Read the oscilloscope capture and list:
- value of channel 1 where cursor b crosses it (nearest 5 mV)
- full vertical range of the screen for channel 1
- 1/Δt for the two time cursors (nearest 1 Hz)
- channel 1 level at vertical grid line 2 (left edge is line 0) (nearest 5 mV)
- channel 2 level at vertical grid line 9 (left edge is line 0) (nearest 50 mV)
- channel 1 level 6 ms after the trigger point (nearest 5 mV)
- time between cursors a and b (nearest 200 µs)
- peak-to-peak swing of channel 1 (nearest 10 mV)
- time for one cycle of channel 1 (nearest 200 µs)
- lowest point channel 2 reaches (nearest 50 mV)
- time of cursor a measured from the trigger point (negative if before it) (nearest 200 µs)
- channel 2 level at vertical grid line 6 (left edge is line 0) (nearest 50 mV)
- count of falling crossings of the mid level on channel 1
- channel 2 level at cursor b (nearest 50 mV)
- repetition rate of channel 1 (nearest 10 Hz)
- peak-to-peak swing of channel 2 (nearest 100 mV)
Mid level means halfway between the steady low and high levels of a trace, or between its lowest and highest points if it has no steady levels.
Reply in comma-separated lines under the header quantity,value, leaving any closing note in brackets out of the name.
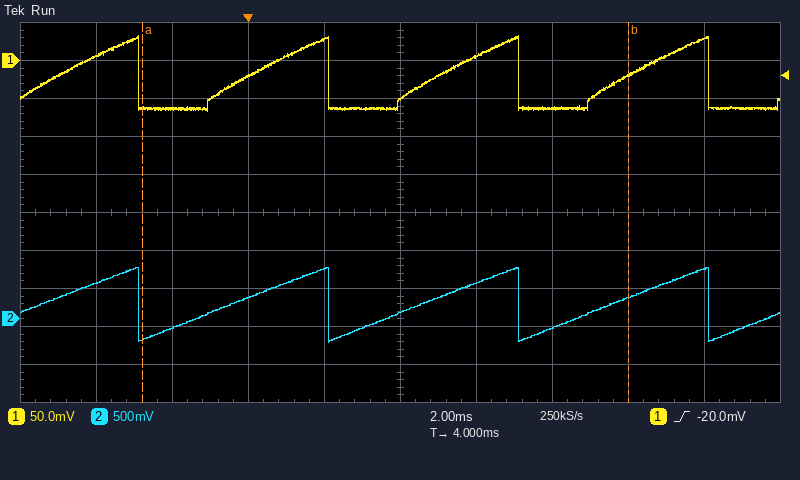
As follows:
quantity,value
value of channel 1 where cursor b crosses it,-20 mV
full vertical range of the screen for channel 1,500 mV
1/Δt for the two time cursors,78 Hz
channel 1 level at vertical grid line 2 (left edge is line 0),-65 mV
channel 2 level at vertical grid line 9 (left edge is line 0),650 mV
channel 1 level 6 ms after the trigger point,5 mV
time between cursors a and b,12.8 ms
peak-to-peak swing of channel 1,100 mV
time for one cycle of channel 1,5.0 ms
lowest point channel 2 reaches,-300 mV
time of cursor a measured from the trigger point (negative if before it),-2.8 ms
channel 2 level at vertical grid line 6 (left edge is line 0),450 mV
count of falling crossings of the mid level on channel 1,4
channel 2 level at cursor b,300 mV
repetition rate of channel 1,200 Hz
peak-to-peak swing of channel 2,1.00 V
